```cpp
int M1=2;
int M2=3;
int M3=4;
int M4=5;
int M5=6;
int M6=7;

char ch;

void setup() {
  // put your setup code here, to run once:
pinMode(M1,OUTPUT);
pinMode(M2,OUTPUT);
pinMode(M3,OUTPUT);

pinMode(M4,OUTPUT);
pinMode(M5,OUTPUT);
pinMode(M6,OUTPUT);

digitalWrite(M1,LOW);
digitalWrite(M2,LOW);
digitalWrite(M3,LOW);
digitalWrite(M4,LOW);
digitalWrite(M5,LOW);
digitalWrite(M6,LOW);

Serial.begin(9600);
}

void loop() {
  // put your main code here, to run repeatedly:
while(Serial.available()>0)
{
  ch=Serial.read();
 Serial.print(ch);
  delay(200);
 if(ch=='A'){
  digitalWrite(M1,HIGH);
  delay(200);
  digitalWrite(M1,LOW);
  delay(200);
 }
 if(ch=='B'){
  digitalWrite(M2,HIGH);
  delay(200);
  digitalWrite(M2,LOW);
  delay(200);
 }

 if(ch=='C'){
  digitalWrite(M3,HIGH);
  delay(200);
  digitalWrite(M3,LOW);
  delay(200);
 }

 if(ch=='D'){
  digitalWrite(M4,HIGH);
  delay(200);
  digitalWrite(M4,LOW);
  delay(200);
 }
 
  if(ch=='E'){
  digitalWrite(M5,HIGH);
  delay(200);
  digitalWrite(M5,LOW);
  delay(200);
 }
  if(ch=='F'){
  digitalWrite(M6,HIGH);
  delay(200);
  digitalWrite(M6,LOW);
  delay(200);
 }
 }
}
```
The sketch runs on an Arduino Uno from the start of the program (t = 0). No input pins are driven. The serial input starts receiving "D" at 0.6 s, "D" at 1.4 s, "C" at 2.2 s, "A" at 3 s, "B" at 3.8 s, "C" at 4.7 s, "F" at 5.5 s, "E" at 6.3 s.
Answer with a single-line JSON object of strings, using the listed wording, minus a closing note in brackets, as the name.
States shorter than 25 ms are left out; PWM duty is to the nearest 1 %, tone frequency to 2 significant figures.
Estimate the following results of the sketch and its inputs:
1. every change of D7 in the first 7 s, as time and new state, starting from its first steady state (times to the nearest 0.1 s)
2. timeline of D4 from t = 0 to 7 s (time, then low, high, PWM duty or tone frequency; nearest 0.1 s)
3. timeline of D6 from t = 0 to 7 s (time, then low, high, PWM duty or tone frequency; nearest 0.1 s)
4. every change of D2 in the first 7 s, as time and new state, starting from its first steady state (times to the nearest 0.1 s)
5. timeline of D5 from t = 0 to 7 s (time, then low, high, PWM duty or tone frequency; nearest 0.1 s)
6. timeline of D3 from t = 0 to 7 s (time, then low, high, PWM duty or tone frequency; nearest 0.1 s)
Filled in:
{"every change of D7 in the first 7 s, as time and new state, starting from its first steady state": "0 s low; 5.7 s high; 5.9 s low", "timeline of D4 from t = 0 to 7 s": "0 s low; 2.4 s high; 2.6 s low; 4.9 s high; 5.1 s low", "timeline of D6 from t = 0 to 7 s": "0 s low; 6.5 s high; 6.7 s low", "every change of D2 in the first 7 s, as time and new state, starting from its first steady state": "0 s low; 3.2 s high; 3.4 s low", "timeline of D5 from t = 0 to 7 s": "0 s low; 0.8 s high; 1 s low; 1.6 s high; 1.8 s low", "timeline of D3 from t = 0 to 7 s": "0 s low; 4 s high; 4.2 s low"}
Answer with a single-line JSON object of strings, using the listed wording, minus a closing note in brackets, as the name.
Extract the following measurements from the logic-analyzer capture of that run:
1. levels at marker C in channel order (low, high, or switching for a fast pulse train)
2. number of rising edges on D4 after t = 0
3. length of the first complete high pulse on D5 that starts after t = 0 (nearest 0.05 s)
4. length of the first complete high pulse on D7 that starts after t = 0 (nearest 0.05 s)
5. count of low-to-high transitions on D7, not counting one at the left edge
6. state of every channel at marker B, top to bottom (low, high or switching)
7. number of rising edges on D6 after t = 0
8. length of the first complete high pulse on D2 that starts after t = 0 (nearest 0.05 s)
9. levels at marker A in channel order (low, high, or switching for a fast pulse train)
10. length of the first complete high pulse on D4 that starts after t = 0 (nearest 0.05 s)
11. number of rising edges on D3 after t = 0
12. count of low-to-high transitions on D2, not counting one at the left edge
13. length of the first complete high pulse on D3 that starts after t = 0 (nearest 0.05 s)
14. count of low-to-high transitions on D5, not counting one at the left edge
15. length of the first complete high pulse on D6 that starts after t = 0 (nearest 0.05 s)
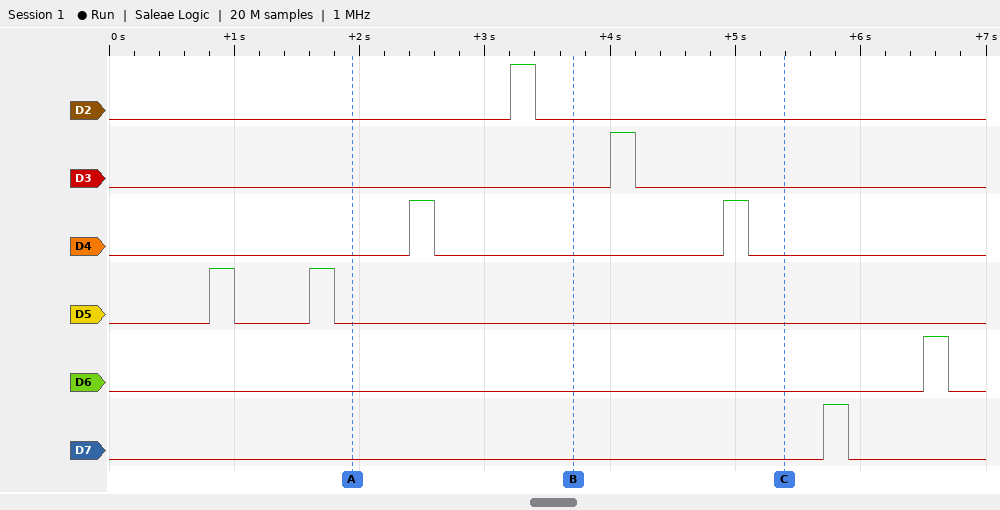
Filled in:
{"levels at marker C in channel order": "D2 low, D3 low, D4 low, D5 low, D6 low, D7 low", "number of rising edges on D4 after t = 0": "2", "length of the first complete high pulse on D5 that starts after t = 0": "0.20 s", "length of the first complete high pulse on D7 that starts after t = 0": "0.20 s", "count of low-to-high transitions on D7, not counting one at the left edge": "1", "state of every channel at marker B, top to bottom": "D2 low, D3 low, D4 low, D5 low, D6 low, D7 low", "number of rising edges on D6 after t = 0": "1", "length of the first complete high pulse on D2 that starts after t = 0": "0.20 s", "levels at marker A in channel order": "D2 low, D3 low, D4 low, D5 low, D6 low, D7 low", "length of the first complete high pulse on D4 that starts after t = 0": "0.20 s", "number of rising edges on D3 after t = 0": "1", "count of low-to-high transitions on D2, not counting one at the left edge": "1", "length of the first complete high pulse on D3 that starts after t = 0": "0.20 s", "count of low-to-high transitions on D5, not counting one at the left edge": "2", "length of the first complete high pulse on D6 that starts after t = 0": "0.20 s"}
